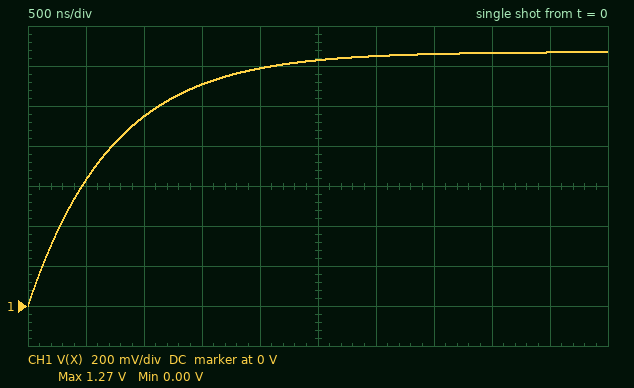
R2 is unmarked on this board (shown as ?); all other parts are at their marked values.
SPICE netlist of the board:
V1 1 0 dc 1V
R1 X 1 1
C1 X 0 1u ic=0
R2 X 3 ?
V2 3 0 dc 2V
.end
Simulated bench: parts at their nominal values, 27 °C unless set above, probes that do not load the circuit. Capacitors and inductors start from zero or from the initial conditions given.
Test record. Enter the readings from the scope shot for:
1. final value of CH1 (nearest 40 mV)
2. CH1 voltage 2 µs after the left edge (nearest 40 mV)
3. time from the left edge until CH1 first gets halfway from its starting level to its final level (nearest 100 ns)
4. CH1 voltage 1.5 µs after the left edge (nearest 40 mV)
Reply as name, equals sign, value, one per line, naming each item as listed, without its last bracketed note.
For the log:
final value of CH1 = 1.28 V
CH1 voltage 2 µs after the left edge = 1.20 V
time from the left edge until CH1 first gets halfway from its starting level to its final level = 500 ns
CH1 voltage 1.5 µs after the left edge = 1.12 V
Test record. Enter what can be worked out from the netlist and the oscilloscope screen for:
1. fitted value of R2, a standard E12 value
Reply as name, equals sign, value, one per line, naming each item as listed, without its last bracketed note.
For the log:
fitted value of R2, a standard E12 value = 2.7 Ω
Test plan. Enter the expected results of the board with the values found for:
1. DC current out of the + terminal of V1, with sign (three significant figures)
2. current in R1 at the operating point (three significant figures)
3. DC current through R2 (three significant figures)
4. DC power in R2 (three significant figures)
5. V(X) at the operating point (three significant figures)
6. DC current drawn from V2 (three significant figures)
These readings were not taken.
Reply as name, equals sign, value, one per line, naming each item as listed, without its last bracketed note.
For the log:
DC current out of the + terminal of V1, with sign = -270 mA
current in R1 at the operating point = 270 mA
DC current through R2 = 270 mA
DC power in R2 = 197 mW
V(X) at the operating point = 1.27 V
DC current drawn from V2 = 270 mA
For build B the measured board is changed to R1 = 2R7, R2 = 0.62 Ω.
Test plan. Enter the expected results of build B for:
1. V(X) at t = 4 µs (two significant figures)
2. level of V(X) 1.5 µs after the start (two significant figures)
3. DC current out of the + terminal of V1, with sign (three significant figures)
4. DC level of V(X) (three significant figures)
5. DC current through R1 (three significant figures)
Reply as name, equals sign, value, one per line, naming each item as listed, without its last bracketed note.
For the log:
V(X) at t = 4 µs = 1.8 V
level of V(X) 1.5 µs after the start = 1.7 V
DC current out of the + terminal of V1, with sign = -301 mA
DC level of V(X) = 1.81 V
DC current through R1 = 301 mA
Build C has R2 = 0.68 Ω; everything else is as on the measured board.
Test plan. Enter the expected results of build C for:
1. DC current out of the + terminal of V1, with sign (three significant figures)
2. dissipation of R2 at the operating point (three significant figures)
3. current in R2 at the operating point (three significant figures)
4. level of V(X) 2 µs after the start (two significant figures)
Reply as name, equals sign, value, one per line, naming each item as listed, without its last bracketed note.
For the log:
DC current out of the + terminal of V1, with sign = -595 mA
dissipation of R2 at the operating point = 241 mW
current in R2 at the operating point = 595 mA
level of V(X) 2 µs after the start = 1.6 V
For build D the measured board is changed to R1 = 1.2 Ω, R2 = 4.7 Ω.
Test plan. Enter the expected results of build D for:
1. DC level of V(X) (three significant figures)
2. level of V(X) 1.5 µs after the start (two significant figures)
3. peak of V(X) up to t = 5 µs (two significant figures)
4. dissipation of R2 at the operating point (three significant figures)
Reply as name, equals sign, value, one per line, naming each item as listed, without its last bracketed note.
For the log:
DC level of V(X) = 1.20 V
level of V(X) 1.5 µs after the start = 950 mV
peak of V(X) up to t = 5 µs = 1.2 V
dissipation of R2 at the operating point = 135 mW
